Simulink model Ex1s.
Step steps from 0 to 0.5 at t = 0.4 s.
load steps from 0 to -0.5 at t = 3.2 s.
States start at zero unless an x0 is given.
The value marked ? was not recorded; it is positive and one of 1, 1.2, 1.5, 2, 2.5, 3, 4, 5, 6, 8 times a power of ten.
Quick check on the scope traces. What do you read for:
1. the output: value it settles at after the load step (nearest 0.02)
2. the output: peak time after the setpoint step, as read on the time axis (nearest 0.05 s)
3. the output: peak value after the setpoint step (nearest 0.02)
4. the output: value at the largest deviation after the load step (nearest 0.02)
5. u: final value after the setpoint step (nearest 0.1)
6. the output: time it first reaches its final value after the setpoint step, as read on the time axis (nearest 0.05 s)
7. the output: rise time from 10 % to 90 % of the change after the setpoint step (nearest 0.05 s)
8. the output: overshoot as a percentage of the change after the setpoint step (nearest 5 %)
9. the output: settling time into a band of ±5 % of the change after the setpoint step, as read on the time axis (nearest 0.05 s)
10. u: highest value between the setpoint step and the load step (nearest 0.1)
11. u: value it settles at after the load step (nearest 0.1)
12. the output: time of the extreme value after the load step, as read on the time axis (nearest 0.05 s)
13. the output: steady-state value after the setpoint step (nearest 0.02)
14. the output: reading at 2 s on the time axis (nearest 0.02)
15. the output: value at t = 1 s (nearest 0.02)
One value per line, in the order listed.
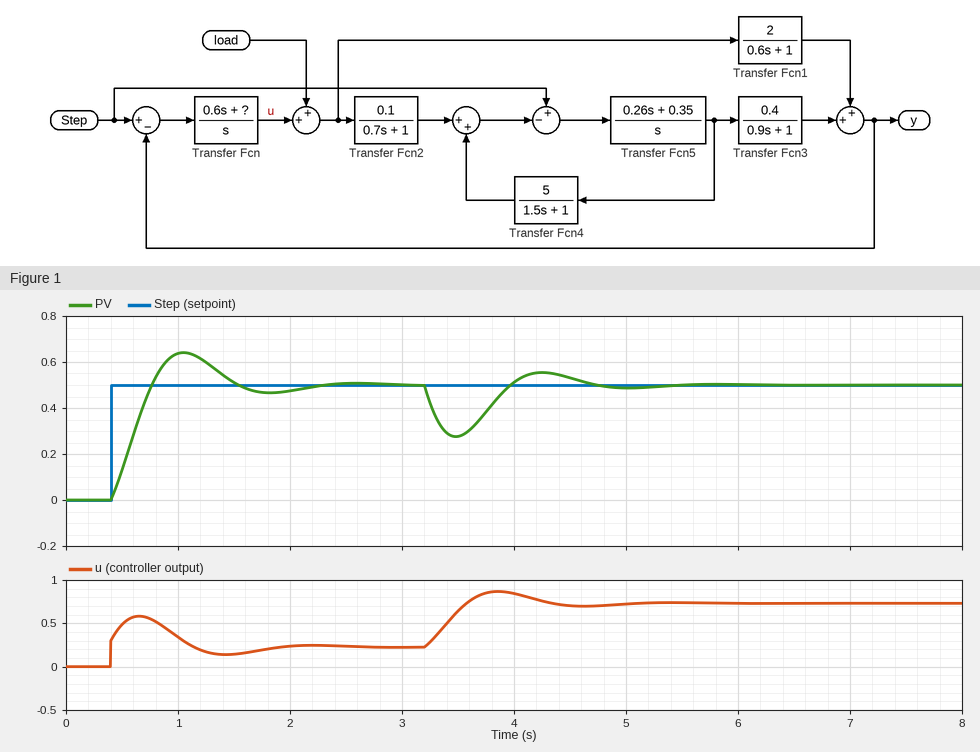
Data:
0.50
1.05 s
0.64
0.28
0.2
0.75 s
0.30 s
30 %
2.00 s
0.6
0.7
3.50 s
0.50
0.48
0.64
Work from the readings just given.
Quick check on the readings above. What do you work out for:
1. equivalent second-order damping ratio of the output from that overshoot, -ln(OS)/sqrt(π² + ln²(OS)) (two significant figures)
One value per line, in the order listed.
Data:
0.36
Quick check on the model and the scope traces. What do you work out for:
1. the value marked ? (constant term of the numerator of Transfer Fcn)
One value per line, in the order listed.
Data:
6
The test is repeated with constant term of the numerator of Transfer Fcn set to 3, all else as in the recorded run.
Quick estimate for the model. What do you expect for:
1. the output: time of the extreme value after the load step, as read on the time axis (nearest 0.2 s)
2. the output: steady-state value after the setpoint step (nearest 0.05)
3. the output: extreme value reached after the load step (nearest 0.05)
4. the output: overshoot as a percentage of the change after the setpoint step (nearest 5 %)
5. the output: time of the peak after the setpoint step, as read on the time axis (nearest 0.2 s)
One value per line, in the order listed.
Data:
3.6 s
0.50
0.25
15 %
1.4 s
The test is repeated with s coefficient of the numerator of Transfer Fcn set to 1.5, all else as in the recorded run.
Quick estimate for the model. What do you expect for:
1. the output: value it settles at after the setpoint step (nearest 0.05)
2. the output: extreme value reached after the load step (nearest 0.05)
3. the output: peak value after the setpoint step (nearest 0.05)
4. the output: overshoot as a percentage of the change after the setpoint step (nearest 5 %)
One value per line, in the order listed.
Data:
0.50
0.35
0.55
10 %
